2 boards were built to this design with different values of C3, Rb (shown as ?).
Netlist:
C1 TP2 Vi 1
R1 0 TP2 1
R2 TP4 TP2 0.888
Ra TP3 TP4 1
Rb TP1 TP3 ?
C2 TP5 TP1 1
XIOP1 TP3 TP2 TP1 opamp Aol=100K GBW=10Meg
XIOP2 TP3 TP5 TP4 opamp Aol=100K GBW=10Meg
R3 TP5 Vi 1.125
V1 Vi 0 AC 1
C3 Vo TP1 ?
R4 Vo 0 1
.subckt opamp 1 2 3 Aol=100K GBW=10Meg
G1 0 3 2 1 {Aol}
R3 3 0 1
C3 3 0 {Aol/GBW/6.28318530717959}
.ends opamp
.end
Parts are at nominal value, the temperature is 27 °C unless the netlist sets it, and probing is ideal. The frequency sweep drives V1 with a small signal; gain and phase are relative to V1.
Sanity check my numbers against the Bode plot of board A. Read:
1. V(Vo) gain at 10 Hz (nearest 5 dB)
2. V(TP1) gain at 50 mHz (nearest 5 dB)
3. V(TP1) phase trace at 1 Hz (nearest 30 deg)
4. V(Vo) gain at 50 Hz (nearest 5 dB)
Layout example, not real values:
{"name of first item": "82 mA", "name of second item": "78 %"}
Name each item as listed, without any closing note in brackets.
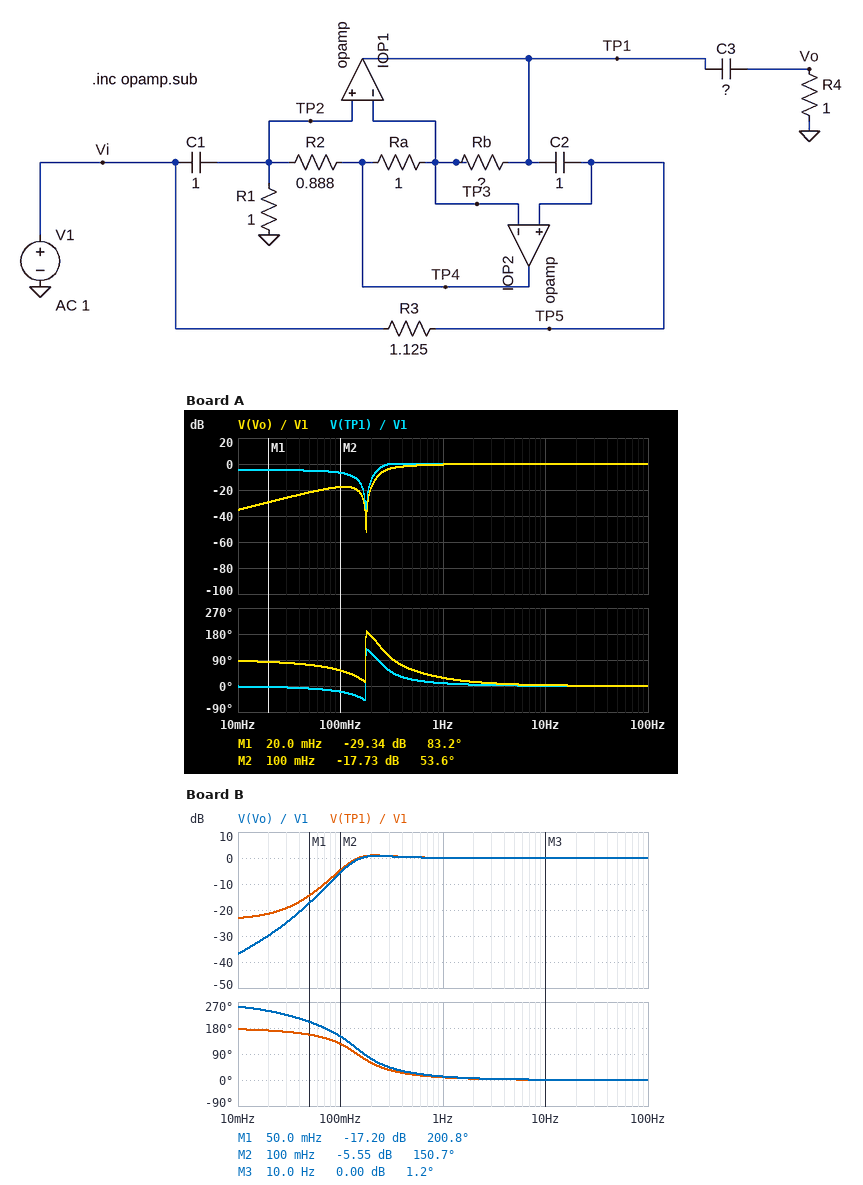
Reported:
{"V(Vo) gain at 10 Hz": "0 dB", "V(TP1) gain at 50 mHz": "-5 dB", "V(TP1) phase trace at 1 Hz": "0 deg", "V(Vo) gain at 50 Hz": "0 dB"}
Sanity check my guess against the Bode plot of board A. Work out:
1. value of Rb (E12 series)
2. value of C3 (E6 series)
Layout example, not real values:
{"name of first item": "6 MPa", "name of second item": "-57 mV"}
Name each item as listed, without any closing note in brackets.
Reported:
{"value of Rb": "0.47 Ω", "value of C3": "470 mF"}
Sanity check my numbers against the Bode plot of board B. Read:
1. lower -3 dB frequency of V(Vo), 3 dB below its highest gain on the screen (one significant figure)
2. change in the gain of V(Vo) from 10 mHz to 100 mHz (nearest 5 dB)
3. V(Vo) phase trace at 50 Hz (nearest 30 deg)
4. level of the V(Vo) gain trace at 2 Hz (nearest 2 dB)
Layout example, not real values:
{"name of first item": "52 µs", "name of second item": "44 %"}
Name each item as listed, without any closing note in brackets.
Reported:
{"lower -3 dB frequency of V(Vo), 3 dB below its highest gain on the screen": "100 mHz", "change in the gain of V(Vo) from 10 mHz to 100 mHz": "30 dB", "V(Vo) phase trace at 50 Hz": "0 deg", "level of the V(Vo) gain trace at 2 Hz": "0 dB"}
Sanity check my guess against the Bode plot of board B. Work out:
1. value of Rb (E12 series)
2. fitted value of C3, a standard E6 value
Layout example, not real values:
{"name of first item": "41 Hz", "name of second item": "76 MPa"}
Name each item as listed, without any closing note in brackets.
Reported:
{"value of Rb": "1.2 Ω", "fitted value of C3, a standard E6 value": "3.3 F"}
